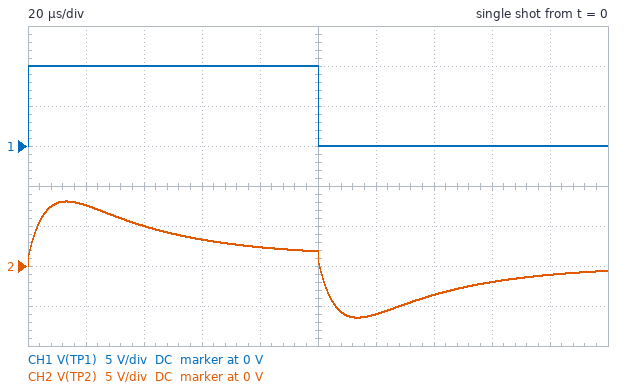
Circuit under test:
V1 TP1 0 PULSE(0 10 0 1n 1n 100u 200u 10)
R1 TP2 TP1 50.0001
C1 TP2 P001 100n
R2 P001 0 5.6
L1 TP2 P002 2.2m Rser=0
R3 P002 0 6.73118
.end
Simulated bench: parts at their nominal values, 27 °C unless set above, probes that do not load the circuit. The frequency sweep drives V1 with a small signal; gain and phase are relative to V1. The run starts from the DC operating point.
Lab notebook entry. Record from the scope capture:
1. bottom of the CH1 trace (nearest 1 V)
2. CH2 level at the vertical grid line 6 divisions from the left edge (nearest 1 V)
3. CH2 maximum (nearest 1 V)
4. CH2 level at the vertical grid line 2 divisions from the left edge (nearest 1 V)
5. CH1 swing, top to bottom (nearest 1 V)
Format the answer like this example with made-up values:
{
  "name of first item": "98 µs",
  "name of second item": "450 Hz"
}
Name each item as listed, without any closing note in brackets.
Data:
{
  "bottom of the CH1 trace": "0 V",
  "CH2 level at the vertical grid line 6 divisions from the left edge": "-6 V",
  "CH2 maximum": "8 V",
  "CH2 level at the vertical grid line 2 divisions from the left edge": "5 V",
  "CH1 swing, top to bottom": "10 V"
}
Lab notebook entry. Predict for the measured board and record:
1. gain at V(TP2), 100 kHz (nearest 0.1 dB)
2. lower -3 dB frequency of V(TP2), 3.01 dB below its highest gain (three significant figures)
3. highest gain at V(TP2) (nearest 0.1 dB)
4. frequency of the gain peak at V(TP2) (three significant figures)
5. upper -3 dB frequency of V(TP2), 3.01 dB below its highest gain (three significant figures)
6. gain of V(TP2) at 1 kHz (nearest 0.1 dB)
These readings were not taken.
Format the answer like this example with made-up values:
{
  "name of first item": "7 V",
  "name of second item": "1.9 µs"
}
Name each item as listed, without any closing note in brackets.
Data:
{
  "gain at V(TP2), 100 kHz": "-10.6 dB",
  "lower -3 dB frequency of V(TP2), 3.01 dB below its highest gain": "3.51 kHz",
  "highest gain at V(TP2)": "-0.2 dB",
  "frequency of the gain peak at V(TP2)": "10.8 kHz",
  "upper -3 dB frequency of V(TP2), 3.01 dB below its highest gain": "33.3 kHz",
  "gain of V(TP2) at 1 kHz": "-11.5 dB"
}
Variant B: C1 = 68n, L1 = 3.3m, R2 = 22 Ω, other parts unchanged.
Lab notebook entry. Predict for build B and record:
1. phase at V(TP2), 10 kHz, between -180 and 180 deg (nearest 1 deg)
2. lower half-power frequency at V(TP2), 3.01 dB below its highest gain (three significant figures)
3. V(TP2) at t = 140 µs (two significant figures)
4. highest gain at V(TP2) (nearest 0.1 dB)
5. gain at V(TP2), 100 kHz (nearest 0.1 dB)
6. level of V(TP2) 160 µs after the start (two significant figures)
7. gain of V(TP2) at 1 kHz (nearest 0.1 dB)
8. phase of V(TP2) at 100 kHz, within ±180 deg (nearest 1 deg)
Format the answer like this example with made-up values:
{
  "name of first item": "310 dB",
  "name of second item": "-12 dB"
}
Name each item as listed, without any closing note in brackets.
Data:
{
  "phase at V(TP2), 10 kHz, between -180 and 180 deg": "2 deg",
  "lower half-power frequency at V(TP2), 3.01 dB below its highest gain": "2.45 kHz",
  "V(TP2) at t = 140 µs": "-4.1 V",
  "highest gain at V(TP2)": "-0.2 dB",
  "gain at V(TP2), 100 kHz": "-7.4 dB",
  "level of V(TP2) 160 µs after the start": "-2.8 V",
  "gain of V(TP2) at 1 kHz": "-8.8 dB",
  "phase of V(TP2) at 100 kHz, within ±180 deg": "-28 deg"
}
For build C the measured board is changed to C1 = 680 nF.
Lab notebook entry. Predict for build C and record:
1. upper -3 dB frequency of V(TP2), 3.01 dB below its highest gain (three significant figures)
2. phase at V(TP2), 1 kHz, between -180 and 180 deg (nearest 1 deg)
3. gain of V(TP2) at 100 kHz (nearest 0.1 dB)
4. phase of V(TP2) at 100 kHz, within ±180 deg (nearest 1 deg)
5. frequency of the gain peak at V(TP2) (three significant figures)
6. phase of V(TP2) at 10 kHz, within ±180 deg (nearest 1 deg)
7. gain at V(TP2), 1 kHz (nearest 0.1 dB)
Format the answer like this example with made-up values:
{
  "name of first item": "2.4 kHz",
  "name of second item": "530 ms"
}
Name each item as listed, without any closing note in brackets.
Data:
{
  "upper -3 dB frequency of V(TP2), 3.01 dB below its highest gain": "7.44 kHz",
  "phase at V(TP2), 1 kHz, between -180 and 180 deg": "48 deg",
  "gain of V(TP2) at 100 kHz": "-19.2 dB",
  "phase of V(TP2) at 100 kHz, within ±180 deg": "-20 deg",
  "frequency of the gain peak at V(TP2)": "4.15 kHz",
  "phase of V(TP2) at 10 kHz, within ±180 deg": "-48 deg",
  "gain at V(TP2), 1 kHz": "-11.2 dB"
}
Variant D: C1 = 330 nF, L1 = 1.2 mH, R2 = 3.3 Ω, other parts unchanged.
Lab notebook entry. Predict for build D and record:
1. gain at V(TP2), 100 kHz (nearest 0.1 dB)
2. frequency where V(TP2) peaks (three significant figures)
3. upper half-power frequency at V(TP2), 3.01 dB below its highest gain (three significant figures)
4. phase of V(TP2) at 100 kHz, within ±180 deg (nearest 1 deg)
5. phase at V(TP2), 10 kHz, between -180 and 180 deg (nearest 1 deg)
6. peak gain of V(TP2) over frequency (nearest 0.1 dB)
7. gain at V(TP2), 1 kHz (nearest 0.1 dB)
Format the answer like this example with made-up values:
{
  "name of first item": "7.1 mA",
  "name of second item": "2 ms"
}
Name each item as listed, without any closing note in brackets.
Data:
{
  "gain at V(TP2), 100 kHz": "-19.2 dB",
  "frequency where V(TP2) peaks": "8.22 kHz",
  "upper half-power frequency at V(TP2), 3.01 dB below its highest gain": "14.9 kHz",
  "phase of V(TP2) at 100 kHz, within ±180 deg": "-50 deg",
  "phase at V(TP2), 10 kHz, between -180 and 180 deg": "-18 deg",
  "peak gain of V(TP2) over frequency": "-1.1 dB",
  "gain at V(TP2), 1 kHz": "-15.0 dB"
}
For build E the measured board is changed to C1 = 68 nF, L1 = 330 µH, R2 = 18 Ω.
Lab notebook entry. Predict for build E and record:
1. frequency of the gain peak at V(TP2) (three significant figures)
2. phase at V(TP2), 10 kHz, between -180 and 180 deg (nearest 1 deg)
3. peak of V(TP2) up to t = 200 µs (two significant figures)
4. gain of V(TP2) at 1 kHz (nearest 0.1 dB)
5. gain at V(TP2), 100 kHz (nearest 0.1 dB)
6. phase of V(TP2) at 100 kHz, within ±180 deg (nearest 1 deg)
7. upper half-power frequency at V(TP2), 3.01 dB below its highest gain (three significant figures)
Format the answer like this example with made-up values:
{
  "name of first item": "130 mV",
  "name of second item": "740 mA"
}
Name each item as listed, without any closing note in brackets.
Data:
{
  "frequency of the gain peak at V(TP2)": "31.4 kHz",
  "phase at V(TP2), 10 kHz, between -180 and 180 deg": "49 deg",
  "peak of V(TP2) up to t = 200 µs": "5.7 V",
  "gain of V(TP2) at 1 kHz": "-18.1 dB",
  "gain at V(TP2), 100 kHz": "-7.3 dB",
  "phase of V(TP2) at 100 kHz, within ±180 deg": "-28 deg",
  "upper half-power frequency at V(TP2), 3.01 dB below its highest gain": "65.6 kHz"
}
